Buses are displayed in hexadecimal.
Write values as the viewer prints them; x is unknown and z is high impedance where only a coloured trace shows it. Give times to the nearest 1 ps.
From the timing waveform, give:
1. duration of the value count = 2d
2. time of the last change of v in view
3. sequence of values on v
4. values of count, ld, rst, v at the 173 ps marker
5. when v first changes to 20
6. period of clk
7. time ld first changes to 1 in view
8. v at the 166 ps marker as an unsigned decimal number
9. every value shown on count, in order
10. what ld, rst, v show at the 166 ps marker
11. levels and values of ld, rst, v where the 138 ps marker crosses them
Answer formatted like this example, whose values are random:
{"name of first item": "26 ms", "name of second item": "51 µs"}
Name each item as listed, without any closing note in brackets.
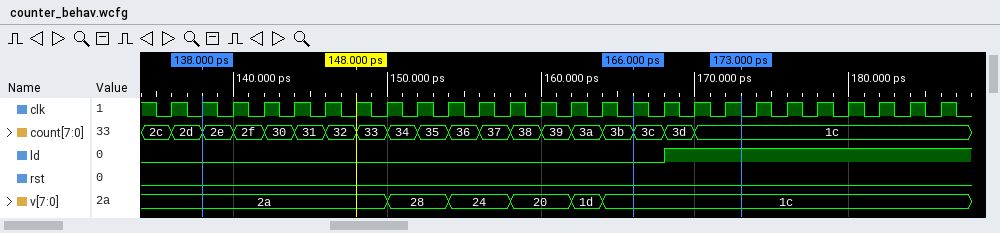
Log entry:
{"duration of the value count = 2d": "2 ps", "time of the last change of v in view": "164 ps", "sequence of values on v": "2a, 28, 24, 20, 1d, 1c", "values of count, ld, rst, v at the 173 ps marker": "count=1c, ld=1, rst=0, v=1c", "when v first changes to 20": "158 ps", "period of clk": "2 ps", "time ld first changes to 1 in view": "168 ps", "v at the 166 ps marker as an unsigned decimal number": "28", "every value shown on count, in order": "2c, 2d, 2e, 2f, 30, 31, 32, 33, 34, 35, 36, 37, 38, 39, 3a, 3b, 3c, 3d, 1c", "what ld, rst, v show at the 166 ps marker": "ld=0, rst=0, v=1c", "levels and values of ld, rst, v where the 138 ps marker crosses them": "ld=0, rst=0, v=2a"}
